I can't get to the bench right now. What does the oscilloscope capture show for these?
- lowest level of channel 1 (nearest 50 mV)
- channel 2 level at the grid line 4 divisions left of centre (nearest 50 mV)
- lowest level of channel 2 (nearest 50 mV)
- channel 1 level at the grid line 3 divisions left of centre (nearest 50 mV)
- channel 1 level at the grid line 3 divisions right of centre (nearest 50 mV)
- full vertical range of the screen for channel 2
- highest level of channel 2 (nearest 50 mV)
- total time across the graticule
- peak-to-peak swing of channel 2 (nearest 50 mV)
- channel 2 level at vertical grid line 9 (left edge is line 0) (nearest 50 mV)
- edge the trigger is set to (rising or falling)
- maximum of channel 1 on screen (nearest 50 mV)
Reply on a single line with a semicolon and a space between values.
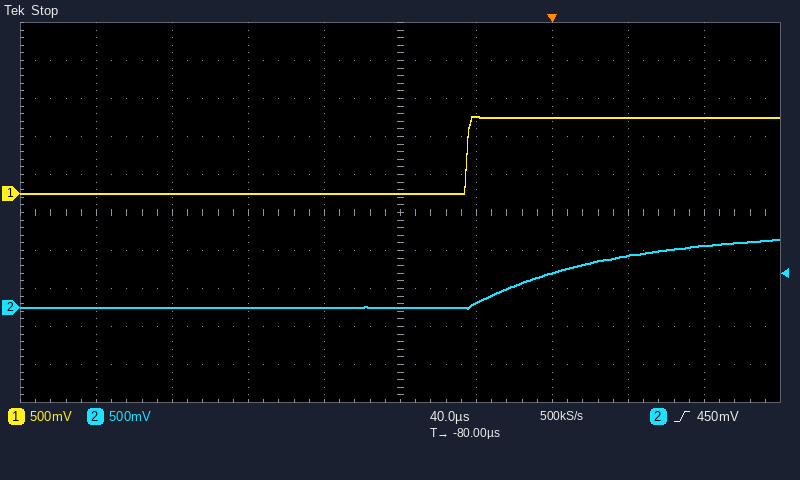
0 mV; 0 mV; 0 mV; 0 mV; 1.00 V; 5 V; 900 mV; 400 µs; 900 mV; 800 mV; rising; 1.00 V
